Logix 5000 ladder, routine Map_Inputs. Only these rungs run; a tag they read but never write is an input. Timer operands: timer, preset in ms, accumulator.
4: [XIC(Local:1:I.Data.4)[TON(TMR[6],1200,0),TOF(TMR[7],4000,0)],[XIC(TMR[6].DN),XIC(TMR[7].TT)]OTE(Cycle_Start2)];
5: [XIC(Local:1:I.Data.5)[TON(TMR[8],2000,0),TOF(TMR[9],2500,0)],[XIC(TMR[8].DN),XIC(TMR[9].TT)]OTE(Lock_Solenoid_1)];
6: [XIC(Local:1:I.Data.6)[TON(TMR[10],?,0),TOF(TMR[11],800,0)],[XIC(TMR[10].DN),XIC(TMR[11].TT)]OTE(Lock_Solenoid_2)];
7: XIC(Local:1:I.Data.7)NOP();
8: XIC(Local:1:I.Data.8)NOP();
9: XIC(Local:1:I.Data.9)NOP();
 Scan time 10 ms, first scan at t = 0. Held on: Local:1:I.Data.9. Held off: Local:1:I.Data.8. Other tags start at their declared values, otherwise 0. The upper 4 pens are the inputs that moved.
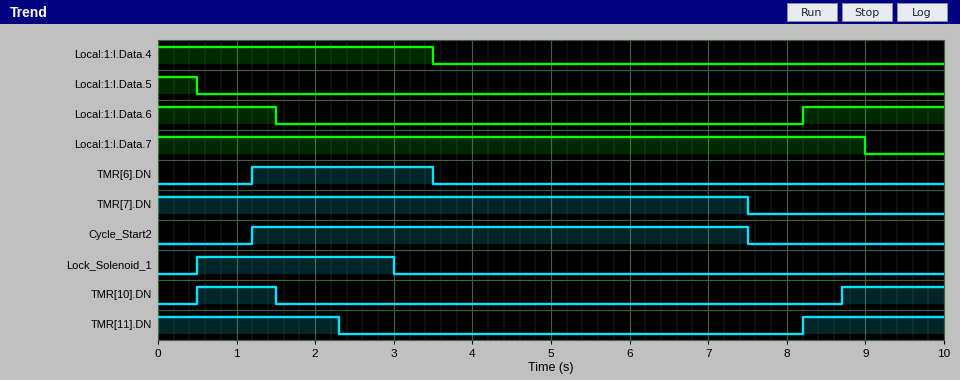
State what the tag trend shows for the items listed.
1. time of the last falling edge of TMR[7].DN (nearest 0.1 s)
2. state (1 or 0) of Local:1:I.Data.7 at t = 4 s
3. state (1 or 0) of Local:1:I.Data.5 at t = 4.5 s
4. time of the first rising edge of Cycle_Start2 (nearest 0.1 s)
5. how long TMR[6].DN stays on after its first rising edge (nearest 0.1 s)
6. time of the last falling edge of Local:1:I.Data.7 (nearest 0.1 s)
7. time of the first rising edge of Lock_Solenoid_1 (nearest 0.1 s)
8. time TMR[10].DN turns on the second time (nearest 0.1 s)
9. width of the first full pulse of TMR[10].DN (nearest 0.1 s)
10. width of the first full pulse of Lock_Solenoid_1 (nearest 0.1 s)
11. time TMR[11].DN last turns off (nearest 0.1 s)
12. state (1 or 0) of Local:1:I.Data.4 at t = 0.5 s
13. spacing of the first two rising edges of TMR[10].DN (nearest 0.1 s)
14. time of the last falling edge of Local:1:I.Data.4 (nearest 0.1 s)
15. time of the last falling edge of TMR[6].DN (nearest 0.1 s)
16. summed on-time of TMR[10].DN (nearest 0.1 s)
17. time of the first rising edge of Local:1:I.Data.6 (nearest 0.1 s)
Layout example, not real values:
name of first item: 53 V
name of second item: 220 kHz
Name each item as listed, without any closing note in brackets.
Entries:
time of the last falling edge of TMR[7].DN: 7.5 s
state (1 or 0) of Local:1:I.Data.7 at t = 4 s: 1
state (1 or 0) of Local:1:I.Data.5 at t = 4.5 s: 0
time of the first rising edge of Cycle_Start2: 1.2 s
how long TMR[6].DN stays on after its first rising edge: 2.3 s
time of the last falling edge of Local:1:I.Data.7: 9.0 s
time of the first rising edge of Lock_Solenoid_1: 0.5 s
time TMR[10].DN turns on the second time: 8.7 s
width of the first full pulse of TMR[10].DN: 1.0 s
width of the first full pulse of Lock_Solenoid_1: 2.5 s
time TMR[11].DN last turns off: 2.3 s
state (1 or 0) of Local:1:I.Data.4 at t = 0.5 s: 1
spacing of the first two rising edges of TMR[10].DN: 8.2 s
time of the last falling edge of Local:1:I.Data.4: 3.5 s
time of the last falling edge of TMR[6].DN: 3.5 s
summed on-time of TMR[10].DN: 2.3 s
time of the first rising edge of Local:1:I.Data.6: 8.2 s
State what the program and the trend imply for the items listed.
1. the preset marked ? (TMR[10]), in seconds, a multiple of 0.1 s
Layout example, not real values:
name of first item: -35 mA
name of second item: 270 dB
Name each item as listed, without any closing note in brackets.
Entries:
the preset marked ? (TMR[10]), in seconds, a multiple of 0.1 s: 0.5 s
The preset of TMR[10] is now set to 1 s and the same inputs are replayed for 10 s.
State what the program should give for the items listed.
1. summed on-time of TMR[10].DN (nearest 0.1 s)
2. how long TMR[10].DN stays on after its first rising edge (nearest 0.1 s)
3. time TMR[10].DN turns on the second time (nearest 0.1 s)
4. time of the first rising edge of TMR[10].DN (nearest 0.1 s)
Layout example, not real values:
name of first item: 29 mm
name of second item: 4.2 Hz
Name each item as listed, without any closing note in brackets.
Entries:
summed on-time of TMR[10].DN: 1.3 s
how long TMR[10].DN stays on after its first rising edge: 0.5 s
time TMR[10].DN turns on the second time: 9.2 s
time of the first rising edge of TMR[10].DN: 1.0 s
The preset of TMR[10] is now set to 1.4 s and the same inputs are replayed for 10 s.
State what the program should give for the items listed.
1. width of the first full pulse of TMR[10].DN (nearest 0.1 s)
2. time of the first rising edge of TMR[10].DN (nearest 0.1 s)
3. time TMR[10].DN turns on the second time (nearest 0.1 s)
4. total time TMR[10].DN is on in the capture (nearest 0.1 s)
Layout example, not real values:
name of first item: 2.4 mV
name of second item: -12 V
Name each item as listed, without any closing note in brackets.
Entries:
width of the first full pulse of TMR[10].DN: 0.1 s
time of the first rising edge of TMR[10].DN: 1.4 s
time TMR[10].DN turns on the second time: 9.6 s
total time TMR[10].DN is on in the capture: 0.5 s
